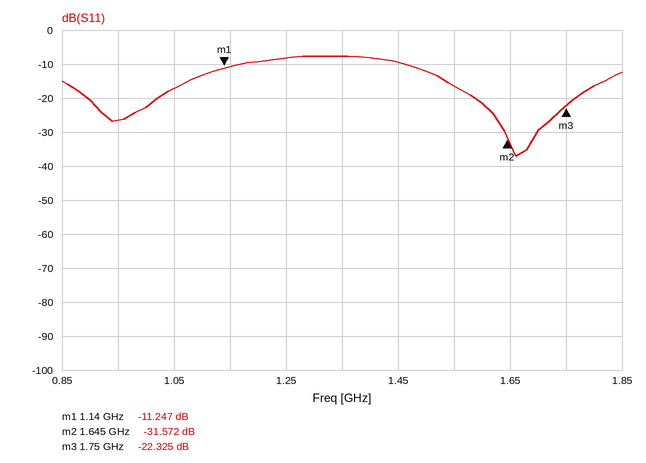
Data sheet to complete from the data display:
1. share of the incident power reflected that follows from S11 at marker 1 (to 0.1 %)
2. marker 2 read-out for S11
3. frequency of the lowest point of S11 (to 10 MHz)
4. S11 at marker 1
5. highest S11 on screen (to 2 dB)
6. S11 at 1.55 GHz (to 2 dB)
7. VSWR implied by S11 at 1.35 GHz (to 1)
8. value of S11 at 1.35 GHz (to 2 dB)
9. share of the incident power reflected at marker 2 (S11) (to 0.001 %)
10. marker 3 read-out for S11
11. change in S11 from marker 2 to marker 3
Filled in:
7.5 %
-31.572 dB
1.66 GHz
-11.247 dB
-8 dB
-16 dB
2
-8 dB
0.070 %
-22.325 dB
9.247 dB
